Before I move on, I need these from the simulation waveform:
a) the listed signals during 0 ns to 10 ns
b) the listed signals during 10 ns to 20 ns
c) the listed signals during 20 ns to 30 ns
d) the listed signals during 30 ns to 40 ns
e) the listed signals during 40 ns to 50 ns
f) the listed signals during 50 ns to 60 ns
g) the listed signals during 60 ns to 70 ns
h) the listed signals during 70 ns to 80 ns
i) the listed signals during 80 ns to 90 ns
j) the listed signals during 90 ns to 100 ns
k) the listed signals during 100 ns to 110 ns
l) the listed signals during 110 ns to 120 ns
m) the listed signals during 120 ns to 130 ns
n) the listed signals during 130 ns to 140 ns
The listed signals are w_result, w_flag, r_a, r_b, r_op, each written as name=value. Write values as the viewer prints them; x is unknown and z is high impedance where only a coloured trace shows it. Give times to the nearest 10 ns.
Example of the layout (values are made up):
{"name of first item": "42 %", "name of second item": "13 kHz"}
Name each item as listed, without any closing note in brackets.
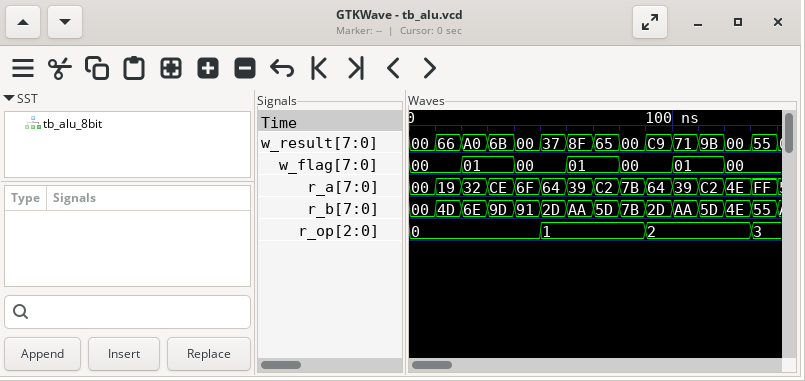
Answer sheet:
{"the listed signals during 0 ns to 10 ns": "w_result=00, w_flag=00, r_a=00, r_b=00, r_op=0", "the listed signals during 10 ns to 20 ns": "w_result=66, w_flag=00, r_a=19, r_b=4D, r_op=0", "the listed signals during 20 ns to 30 ns": "w_result=A0, w_flag=01, r_a=32, r_b=6E, r_op=0", "the listed signals during 30 ns to 40 ns": "w_result=6B, w_flag=01, r_a=CE, r_b=9D, r_op=0", "the listed signals during 40 ns to 50 ns": "w_result=00, w_flag=00, r_a=6F, r_b=91, r_op=0", "the listed signals during 50 ns to 60 ns": "w_result=37, w_flag=00, r_a=64, r_b=2D, r_op=1", "the listed signals during 60 ns to 70 ns": "w_result=8F, w_flag=01, r_a=39, r_b=AA, r_op=1", "the listed signals during 70 ns to 80 ns": "w_result=65, w_flag=01, r_a=C2, r_b=5D, r_op=1", "the listed signals during 80 ns to 90 ns": "w_result=00, w_flag=00, r_a=7B, r_b=7B, r_op=1", "the listed signals during 90 ns to 100 ns": "w_result=C9, w_flag=00, r_a=64, r_b=2D, r_op=2", "the listed signals during 100 ns to 110 ns": "w_result=71, w_flag=01, r_a=39, r_b=AA, r_op=2", "the listed signals during 110 ns to 120 ns": "w_result=9B, w_flag=01, r_a=C2, r_b=5D, r_op=2", "the listed signals during 120 ns to 130 ns": "w_result=00, w_flag=00, r_a=4E, r_b=4E, r_op=2", "the listed signals during 130 ns to 140 ns": "w_result=55, w_flag=00, r_a=FF, r_b=55, r_op=3"}
